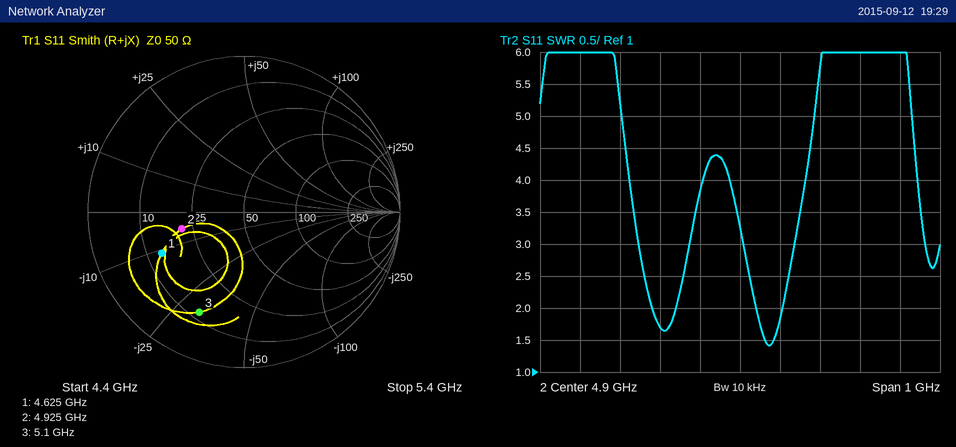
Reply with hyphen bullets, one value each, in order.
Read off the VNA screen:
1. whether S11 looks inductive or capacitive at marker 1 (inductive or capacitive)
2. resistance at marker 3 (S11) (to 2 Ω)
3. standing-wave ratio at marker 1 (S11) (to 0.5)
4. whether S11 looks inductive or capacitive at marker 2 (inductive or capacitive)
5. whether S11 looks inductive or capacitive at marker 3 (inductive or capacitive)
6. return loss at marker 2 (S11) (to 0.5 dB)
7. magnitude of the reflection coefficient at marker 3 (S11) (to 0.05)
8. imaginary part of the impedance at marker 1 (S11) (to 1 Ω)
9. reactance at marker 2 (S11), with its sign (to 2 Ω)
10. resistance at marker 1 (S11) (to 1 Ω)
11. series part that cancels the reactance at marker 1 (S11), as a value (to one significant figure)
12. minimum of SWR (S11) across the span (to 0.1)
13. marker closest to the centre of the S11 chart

- capacitive
- 12 Ω
- 4.0
- capacitive
- capacitive
- 7.5 dB
- 0.70
- -11 Ω
- -6 Ω
- 14 Ω
- 400 pH
- 1.4
- marker 2
